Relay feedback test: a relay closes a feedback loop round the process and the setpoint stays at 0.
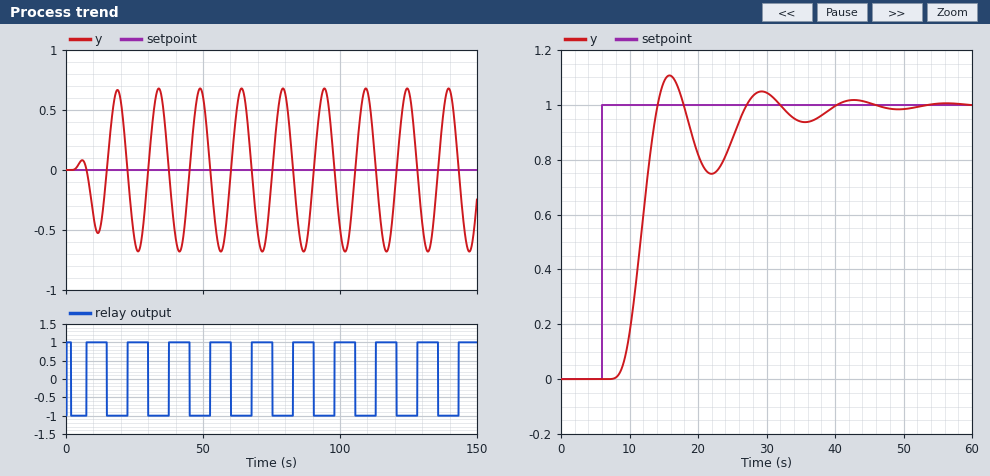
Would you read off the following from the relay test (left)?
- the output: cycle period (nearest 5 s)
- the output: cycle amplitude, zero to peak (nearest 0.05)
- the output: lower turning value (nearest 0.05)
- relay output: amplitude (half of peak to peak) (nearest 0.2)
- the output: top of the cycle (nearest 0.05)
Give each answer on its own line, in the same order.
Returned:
15 s
0.70
-0.70
1.0
0.70
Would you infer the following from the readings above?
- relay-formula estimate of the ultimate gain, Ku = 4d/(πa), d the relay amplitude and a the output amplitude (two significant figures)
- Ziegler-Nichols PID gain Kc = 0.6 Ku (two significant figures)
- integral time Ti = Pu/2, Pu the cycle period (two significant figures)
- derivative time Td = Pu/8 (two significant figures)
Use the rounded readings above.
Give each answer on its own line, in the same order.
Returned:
1.8
1.1
7.5 s
1.9 s
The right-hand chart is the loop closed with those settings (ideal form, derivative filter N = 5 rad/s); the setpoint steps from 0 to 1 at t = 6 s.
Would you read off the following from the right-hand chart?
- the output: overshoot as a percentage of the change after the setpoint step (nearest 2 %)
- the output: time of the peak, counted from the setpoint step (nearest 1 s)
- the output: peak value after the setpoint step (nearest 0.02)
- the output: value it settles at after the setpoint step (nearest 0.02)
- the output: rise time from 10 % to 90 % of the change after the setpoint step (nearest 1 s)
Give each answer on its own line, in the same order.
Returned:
10 %
10 s
1.10
1.00
4 s
